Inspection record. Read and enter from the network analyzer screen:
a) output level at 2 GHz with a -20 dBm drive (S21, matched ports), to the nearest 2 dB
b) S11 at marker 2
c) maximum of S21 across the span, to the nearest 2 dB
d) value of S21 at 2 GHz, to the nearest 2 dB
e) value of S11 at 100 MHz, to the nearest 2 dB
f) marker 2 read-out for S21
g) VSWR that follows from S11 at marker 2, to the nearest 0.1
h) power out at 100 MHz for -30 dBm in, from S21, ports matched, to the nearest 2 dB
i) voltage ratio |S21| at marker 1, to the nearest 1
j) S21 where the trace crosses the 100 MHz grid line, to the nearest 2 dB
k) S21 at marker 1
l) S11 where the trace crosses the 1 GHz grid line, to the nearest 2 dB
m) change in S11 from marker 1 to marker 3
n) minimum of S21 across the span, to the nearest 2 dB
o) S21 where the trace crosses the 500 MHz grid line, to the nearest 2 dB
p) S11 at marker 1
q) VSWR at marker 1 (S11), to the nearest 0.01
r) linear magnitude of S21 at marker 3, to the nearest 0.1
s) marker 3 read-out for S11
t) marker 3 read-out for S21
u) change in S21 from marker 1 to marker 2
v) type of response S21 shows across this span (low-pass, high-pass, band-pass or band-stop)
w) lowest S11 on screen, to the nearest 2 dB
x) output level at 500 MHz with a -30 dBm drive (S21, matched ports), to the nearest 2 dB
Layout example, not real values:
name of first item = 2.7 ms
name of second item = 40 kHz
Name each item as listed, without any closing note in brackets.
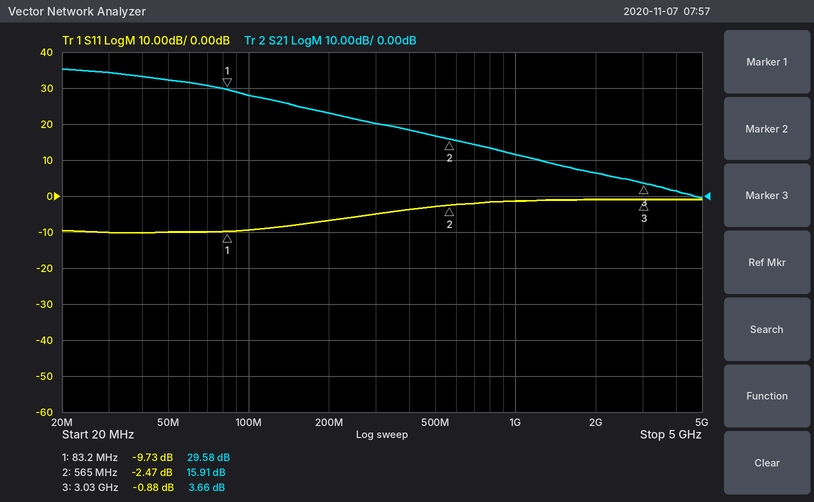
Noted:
output level at 2 GHz with a -20 dBm drive (S21, matched ports), to the nearest 2 dB = -14 dBm
S11 at marker 2 = -2.47 dB
maximum of S21 across the span, to the nearest 2 dB = 36 dB
value of S21 at 2 GHz, to the nearest 2 dB = 6 dB
value of S11 at 100 MHz, to the nearest 2 dB = -10 dB
marker 2 read-out for S21 = 15.91 dB
VSWR that follows from S11 at marker 2, to the nearest 0.1 = 7.1
power out at 100 MHz for -30 dBm in, from S21, ports matched, to the nearest 2 dB = -2 dBm
voltage ratio |S21| at marker 1, to the nearest 1 = 30
S21 where the trace crosses the 100 MHz grid line, to the nearest 2 dB = 28 dB
S21 at marker 1 = 29.58 dB
S11 where the trace crosses the 1 GHz grid line, to the nearest 2 dB = -2 dB
change in S11 from marker 1 to marker 3 = 8.85 dB
minimum of S21 across the span, to the nearest 2 dB = 0 dB
S21 where the trace crosses the 500 MHz grid line, to the nearest 2 dB = 16 dB
S11 at marker 1 = -9.73 dB
VSWR at marker 1 (S11), to the nearest 0.01 = 1.97
linear magnitude of S21 at marker 3, to the nearest 0.1 = 1.5
marker 3 read-out for S11 = -0.88 dB
marker 3 read-out for S21 = 3.66 dB
change in S21 from marker 1 to marker 2 = -13.67 dB
type of response S21 shows across this span = low-pass
lowest S11 on screen, to the nearest 2 dB = -10 dB
output level at 500 MHz with a -30 dBm drive (S21, matched ports), to the nearest 2 dB = -14 dBm
